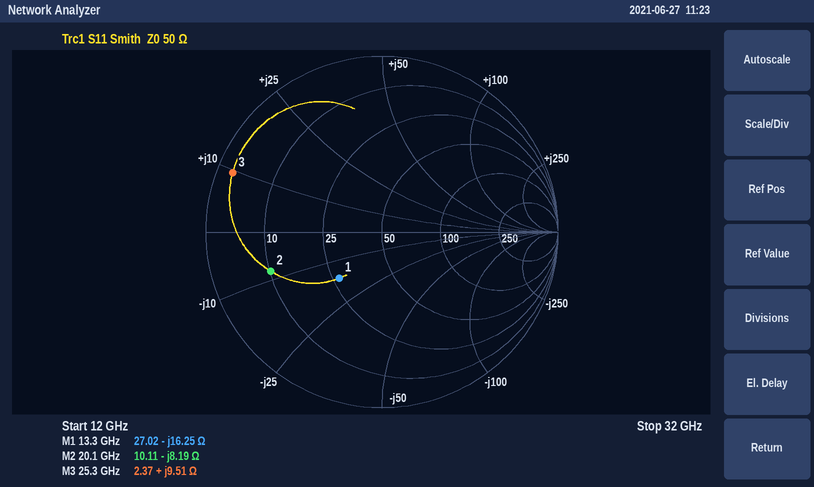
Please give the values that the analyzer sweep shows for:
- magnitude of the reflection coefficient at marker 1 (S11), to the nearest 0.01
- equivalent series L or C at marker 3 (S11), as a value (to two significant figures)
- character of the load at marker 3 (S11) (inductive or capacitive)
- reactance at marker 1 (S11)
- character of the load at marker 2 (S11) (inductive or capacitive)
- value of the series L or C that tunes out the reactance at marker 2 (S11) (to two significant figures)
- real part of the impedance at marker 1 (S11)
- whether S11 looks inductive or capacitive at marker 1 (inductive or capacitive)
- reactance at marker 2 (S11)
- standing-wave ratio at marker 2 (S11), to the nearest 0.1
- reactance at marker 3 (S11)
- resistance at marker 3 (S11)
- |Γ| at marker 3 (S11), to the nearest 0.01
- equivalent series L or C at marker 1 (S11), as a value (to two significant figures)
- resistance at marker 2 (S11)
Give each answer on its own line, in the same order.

0.36
60 pH
inductive
-16.25 Ω
capacitive
65 pH
27.02 Ω
capacitive
-8.19 Ω
5.1
+9.51 Ω
2.37 Ω
0.91
740 fF
10.11 Ω
